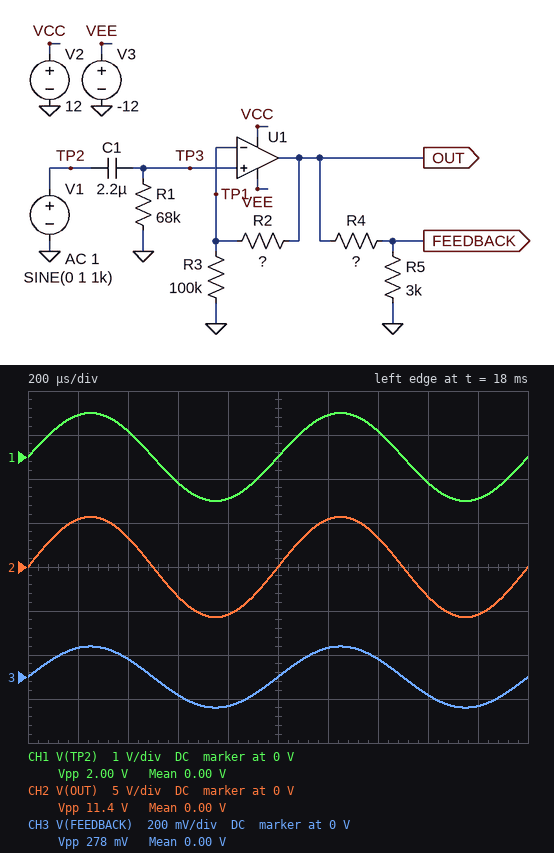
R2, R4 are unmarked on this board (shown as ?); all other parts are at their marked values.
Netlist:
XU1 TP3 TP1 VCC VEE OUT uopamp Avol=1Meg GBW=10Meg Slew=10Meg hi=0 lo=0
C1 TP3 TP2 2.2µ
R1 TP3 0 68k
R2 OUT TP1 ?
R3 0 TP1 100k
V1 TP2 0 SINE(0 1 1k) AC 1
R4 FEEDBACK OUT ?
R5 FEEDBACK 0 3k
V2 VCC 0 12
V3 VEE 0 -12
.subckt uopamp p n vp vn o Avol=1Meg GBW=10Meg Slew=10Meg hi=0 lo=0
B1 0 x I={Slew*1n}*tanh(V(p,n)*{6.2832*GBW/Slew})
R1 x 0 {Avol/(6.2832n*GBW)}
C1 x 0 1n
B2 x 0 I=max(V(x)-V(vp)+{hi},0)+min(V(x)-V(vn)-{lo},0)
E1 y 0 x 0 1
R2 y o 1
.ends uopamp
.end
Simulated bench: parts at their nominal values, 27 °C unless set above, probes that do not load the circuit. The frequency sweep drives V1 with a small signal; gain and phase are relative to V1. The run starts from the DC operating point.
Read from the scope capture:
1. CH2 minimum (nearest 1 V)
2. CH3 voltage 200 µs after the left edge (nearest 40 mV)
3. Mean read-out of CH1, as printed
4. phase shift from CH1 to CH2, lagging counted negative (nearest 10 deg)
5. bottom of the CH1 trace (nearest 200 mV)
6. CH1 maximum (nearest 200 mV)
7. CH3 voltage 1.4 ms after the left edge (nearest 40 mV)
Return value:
-6 V
120 mV
0.00 V
0 deg
-1.0 V
1.0 V
80 mV
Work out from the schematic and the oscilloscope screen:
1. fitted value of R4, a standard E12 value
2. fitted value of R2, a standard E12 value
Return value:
120 kΩ
470 kΩ
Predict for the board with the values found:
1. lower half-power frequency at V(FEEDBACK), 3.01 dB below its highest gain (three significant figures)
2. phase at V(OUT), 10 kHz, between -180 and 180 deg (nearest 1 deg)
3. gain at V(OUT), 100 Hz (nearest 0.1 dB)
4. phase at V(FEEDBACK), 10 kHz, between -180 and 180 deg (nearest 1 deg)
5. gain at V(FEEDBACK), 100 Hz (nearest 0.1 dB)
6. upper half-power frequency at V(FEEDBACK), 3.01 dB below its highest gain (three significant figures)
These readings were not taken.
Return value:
1.06 Hz
0 deg
15.1 dB
0 deg
-17.1 dB
1.75 MHz
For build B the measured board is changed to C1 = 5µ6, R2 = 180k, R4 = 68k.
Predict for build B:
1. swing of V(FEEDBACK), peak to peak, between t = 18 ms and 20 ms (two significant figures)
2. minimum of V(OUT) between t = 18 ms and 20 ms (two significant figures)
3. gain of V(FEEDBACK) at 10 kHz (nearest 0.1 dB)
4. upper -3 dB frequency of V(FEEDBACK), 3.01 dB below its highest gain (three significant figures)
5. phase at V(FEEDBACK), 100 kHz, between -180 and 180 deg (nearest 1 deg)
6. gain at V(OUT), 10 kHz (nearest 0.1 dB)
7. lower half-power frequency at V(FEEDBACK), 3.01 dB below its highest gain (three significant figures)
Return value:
240 mV
-2.8 V
-18.5 dB
3.57 MHz
-2 deg
8.9 dB
418 mHz
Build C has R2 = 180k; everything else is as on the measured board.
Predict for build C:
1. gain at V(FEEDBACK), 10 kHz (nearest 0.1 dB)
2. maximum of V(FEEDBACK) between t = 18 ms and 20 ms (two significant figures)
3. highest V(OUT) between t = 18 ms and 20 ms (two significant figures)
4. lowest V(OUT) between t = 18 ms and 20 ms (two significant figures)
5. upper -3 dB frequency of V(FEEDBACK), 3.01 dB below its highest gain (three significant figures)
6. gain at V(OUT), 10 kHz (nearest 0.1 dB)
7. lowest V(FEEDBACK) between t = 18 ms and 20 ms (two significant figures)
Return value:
-23.3 dB
68 mV
2.8 V
-2.8 V
3.57 MHz
8.9 dB
-68 mV
